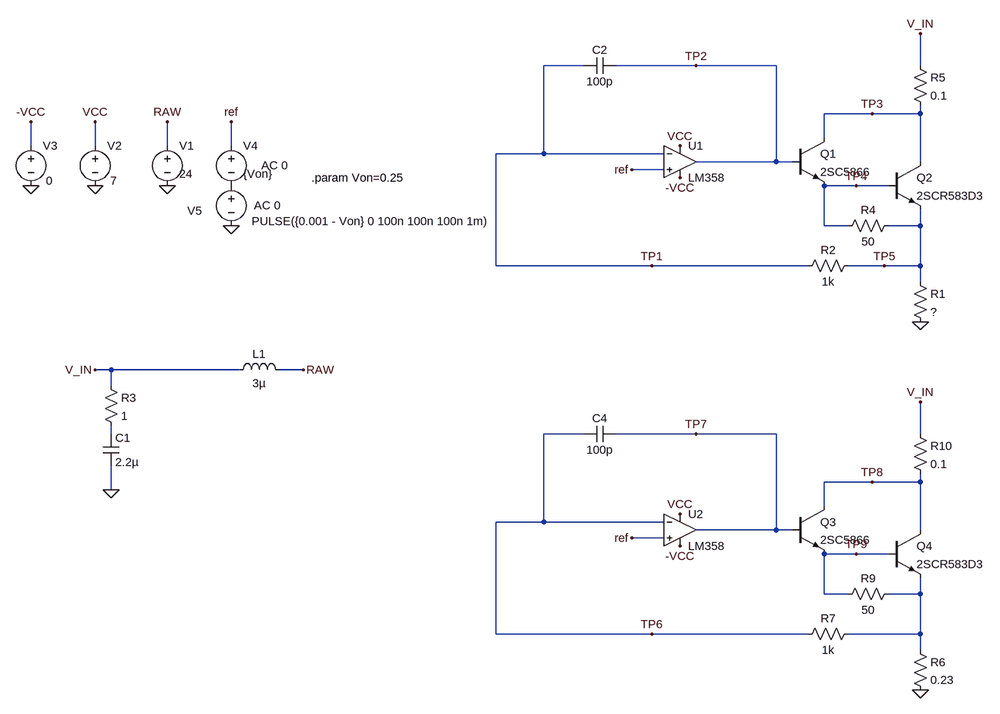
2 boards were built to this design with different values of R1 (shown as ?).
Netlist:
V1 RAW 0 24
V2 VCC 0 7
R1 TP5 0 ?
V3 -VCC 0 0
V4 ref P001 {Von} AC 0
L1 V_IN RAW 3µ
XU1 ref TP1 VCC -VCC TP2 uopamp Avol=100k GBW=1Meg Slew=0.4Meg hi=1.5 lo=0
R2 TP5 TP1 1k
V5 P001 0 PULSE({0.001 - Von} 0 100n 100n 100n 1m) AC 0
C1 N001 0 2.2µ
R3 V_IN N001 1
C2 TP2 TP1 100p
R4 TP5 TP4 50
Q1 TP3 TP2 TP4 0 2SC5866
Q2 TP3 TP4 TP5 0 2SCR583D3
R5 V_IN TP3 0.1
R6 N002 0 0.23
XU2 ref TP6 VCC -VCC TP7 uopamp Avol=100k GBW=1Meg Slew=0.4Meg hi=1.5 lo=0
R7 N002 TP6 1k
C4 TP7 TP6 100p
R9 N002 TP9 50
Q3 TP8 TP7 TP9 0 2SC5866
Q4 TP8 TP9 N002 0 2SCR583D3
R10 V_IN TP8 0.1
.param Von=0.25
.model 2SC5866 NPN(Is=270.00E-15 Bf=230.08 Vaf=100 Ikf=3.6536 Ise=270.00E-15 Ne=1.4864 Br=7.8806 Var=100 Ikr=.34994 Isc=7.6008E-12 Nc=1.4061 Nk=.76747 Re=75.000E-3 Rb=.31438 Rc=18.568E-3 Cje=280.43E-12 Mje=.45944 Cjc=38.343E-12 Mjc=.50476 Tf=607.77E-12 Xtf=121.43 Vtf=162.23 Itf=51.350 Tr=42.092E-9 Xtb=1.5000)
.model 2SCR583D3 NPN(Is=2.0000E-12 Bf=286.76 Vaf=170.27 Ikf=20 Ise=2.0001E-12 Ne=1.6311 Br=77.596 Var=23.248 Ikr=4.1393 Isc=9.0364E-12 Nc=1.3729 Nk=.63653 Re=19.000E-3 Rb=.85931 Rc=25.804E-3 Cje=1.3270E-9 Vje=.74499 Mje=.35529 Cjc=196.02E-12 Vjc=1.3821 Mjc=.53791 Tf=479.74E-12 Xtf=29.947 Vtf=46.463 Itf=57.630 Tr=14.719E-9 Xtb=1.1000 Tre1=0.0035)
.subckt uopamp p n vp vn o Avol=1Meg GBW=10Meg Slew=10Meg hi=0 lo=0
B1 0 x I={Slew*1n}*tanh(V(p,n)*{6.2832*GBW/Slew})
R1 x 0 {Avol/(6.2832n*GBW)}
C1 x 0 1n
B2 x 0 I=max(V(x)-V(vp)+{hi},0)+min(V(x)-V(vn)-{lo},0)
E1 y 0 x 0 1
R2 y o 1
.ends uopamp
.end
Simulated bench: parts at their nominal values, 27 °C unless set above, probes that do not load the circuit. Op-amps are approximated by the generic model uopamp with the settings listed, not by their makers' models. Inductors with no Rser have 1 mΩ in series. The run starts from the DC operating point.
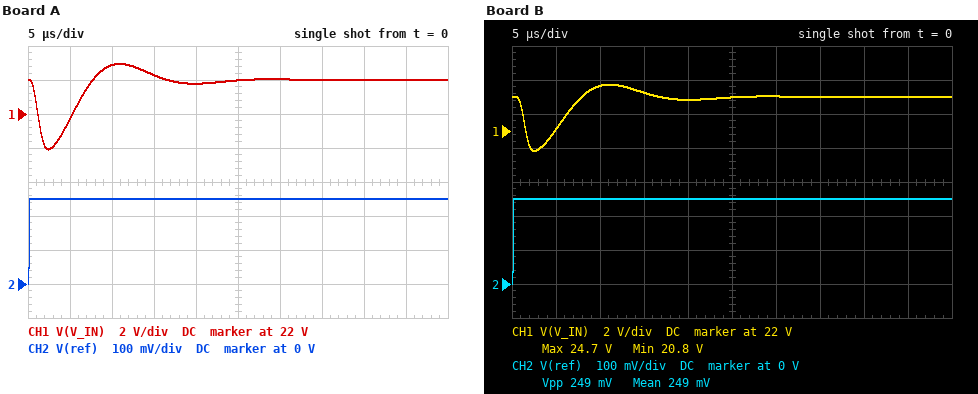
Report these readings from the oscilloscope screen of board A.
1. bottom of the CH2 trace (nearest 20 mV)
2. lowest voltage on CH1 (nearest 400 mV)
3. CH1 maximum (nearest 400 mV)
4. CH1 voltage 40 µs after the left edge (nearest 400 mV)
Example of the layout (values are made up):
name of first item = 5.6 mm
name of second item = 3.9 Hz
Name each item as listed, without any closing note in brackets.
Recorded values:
bottom of the CH2 trace = 0 V
lowest voltage on CH1 = 20.0 V
CH1 maximum = 24.8 V
CH1 voltage 40 µs after the left edge = 24.0 V
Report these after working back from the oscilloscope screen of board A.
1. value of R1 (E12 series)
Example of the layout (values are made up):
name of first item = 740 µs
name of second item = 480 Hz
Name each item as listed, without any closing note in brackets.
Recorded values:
value of R1 = 0.082 Ω
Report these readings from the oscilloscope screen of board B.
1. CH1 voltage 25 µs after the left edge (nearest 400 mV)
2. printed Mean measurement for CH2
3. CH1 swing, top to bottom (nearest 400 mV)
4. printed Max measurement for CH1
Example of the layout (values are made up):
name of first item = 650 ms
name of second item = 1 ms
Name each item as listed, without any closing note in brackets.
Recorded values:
CH1 voltage 25 µs after the left edge = 24.0 V
printed Mean measurement for CH2 = 249 mV
CH1 swing, top to bottom = 4.0 V
printed Max measurement for CH1 = 24.7 V
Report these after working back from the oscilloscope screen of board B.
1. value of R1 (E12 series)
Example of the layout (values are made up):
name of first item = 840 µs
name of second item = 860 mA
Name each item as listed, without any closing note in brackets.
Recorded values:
value of R1 = 0.12 Ω
